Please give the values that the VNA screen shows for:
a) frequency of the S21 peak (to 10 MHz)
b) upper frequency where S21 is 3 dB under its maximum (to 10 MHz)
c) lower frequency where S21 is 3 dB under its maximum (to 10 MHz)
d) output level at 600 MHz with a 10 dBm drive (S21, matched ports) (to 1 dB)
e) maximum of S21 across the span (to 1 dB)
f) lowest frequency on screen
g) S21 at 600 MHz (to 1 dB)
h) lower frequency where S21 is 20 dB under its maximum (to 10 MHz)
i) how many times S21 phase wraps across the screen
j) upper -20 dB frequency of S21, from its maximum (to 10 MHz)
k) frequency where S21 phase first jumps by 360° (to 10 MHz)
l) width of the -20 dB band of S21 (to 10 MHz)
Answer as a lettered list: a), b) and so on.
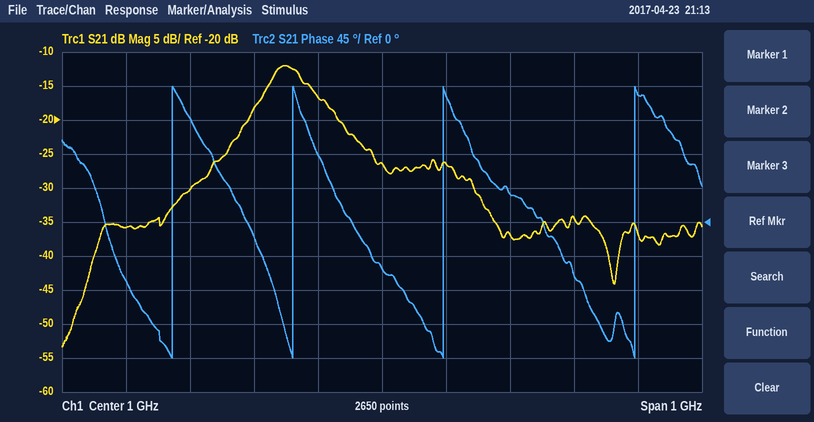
a) 850 MHz
b) 890 MHz
c) 820 MHz
d) -26 dBm
e) -12 dB
f) 500 MHz
g) -36 dB
h) 680 MHz
i) 4
j) 1.16 GHz
k) 670 MHz
l) 480 MHz
